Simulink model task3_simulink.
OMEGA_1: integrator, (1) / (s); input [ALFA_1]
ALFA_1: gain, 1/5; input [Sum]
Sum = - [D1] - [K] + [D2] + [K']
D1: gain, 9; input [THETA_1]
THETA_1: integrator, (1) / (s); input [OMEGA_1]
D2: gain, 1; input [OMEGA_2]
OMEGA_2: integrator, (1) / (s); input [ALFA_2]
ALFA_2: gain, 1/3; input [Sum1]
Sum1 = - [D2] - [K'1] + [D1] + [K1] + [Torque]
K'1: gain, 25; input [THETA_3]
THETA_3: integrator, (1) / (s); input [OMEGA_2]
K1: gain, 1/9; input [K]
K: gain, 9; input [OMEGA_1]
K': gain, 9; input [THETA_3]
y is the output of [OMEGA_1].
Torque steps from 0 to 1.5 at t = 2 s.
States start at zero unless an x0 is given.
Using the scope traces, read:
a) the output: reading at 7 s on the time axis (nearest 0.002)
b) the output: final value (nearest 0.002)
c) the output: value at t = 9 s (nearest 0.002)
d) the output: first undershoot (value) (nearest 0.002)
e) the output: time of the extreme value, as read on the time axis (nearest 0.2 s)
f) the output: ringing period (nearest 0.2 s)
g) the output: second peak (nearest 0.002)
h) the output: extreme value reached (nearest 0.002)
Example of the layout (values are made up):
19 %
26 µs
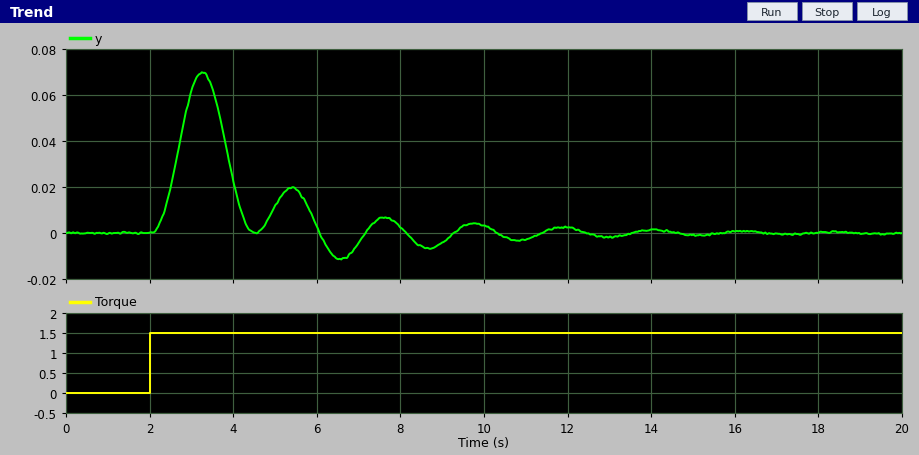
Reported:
-0.004
0.000
-0.004
0.000
3.2 s
2.2 s
0.020
0.070
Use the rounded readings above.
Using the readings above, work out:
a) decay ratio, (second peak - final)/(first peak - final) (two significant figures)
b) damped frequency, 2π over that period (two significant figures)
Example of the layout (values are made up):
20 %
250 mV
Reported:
0.29
2.9 rad/s
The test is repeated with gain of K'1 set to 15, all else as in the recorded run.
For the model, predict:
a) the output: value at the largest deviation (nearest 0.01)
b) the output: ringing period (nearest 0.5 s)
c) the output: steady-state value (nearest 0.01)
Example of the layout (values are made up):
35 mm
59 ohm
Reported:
0.12
2.5 s
0.00
